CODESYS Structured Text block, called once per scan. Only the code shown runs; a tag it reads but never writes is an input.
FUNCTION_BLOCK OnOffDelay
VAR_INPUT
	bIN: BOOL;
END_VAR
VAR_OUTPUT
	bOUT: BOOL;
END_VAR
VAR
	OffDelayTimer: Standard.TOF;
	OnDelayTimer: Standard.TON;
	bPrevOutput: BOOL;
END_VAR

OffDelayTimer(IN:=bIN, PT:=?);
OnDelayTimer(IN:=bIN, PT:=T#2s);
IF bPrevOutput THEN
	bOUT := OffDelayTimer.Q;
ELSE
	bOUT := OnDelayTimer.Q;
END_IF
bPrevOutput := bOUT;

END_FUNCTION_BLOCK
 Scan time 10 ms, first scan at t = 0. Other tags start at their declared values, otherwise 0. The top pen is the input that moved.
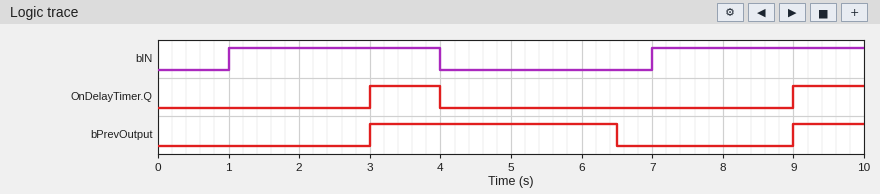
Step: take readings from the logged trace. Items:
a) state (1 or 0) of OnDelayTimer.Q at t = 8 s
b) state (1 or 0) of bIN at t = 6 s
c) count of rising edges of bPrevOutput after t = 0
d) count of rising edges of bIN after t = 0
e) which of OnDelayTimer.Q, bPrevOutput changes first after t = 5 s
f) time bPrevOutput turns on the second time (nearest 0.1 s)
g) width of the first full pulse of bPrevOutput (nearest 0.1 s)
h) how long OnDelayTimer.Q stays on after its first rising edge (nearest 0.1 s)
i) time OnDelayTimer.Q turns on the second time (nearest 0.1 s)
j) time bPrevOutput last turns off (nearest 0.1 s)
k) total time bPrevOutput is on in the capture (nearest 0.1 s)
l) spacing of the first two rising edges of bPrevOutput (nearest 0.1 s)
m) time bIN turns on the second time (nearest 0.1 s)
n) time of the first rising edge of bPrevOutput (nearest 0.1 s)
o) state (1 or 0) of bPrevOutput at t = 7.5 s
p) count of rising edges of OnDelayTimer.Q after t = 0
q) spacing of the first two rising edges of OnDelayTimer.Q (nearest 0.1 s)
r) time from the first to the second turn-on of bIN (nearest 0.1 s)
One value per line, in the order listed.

0
0
2
2
bPrevOutput
9.0 s
3.5 s
1.0 s
9.0 s
6.5 s
4.5 s
6.0 s
7.0 s
3.0 s
0
2
6.0 s
6.0 s
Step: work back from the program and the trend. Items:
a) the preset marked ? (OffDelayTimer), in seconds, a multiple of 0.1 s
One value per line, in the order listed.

2.5 s
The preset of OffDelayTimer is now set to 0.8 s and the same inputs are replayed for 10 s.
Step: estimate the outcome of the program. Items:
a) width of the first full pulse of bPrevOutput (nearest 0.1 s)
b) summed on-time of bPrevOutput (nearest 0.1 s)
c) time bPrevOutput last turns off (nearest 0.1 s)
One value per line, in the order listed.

1.8 s
2.8 s
4.8 s
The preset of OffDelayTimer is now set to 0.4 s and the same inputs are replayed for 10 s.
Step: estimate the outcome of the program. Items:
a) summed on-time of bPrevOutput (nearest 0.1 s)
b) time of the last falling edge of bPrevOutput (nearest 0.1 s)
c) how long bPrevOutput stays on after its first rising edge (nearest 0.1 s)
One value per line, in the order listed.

2.4 s
4.4 s
1.4 s
